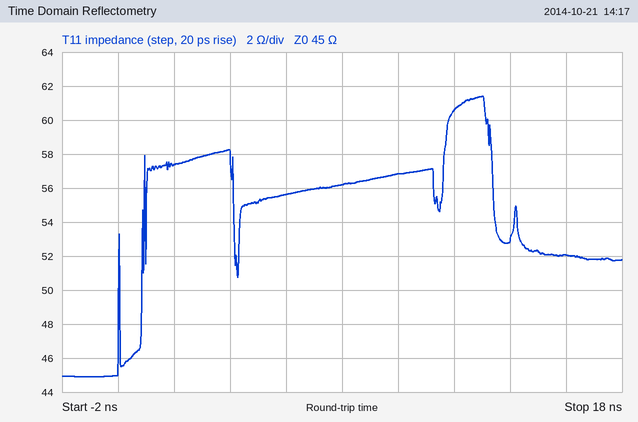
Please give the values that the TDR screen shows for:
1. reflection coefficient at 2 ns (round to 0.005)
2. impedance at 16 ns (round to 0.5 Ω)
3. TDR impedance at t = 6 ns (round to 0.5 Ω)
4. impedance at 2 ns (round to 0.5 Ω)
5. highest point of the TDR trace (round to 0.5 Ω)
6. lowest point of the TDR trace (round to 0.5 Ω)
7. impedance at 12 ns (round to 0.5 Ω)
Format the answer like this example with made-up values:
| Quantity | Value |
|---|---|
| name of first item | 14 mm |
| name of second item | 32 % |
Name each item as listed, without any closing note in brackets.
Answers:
| Quantity | Value |
|---|---|
| reflection coefficient at 2 ns | +0.120 |
| impedance at 16 ns | 52.0 Ω |
| TDR impedance at t = 6 ns | 55.5 Ω |
| impedance at 2 ns | 57.5 Ω |
| highest point of the TDR trace | 61.5 Ω |
| lowest point of the TDR trace | 45.0 Ω |
| impedance at 12 ns | 60.5 Ω |
